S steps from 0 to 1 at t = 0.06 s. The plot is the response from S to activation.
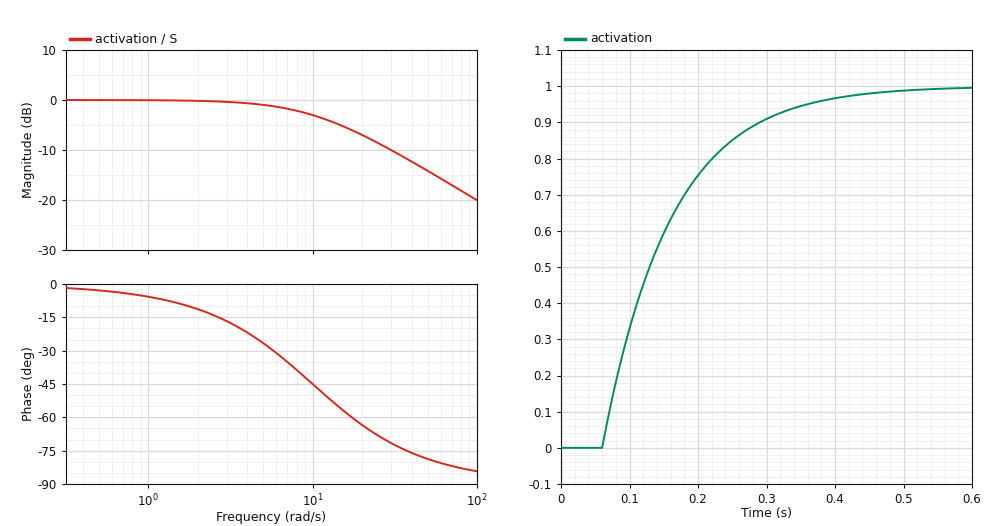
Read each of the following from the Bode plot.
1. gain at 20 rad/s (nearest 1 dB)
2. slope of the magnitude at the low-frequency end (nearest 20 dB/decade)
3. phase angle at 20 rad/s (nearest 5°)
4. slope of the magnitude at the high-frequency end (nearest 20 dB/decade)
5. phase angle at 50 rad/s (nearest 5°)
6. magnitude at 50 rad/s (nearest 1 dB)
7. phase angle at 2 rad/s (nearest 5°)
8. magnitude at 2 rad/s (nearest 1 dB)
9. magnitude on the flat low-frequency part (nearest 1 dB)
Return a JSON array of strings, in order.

["-7 dB", "0 dB/decade", "-65°", "-20 dB/decade", "-80°", "-14 dB", "-10°", "0 dB", "0 dB"]
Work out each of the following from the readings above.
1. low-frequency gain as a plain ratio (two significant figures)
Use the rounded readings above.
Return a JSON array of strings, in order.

["1.0"]
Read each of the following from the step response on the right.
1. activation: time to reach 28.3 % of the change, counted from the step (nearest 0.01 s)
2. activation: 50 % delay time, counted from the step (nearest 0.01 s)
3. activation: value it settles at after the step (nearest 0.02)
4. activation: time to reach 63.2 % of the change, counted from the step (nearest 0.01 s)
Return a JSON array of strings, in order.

["0.03 s", "0.07 s", "1.00", "0.10 s"]
